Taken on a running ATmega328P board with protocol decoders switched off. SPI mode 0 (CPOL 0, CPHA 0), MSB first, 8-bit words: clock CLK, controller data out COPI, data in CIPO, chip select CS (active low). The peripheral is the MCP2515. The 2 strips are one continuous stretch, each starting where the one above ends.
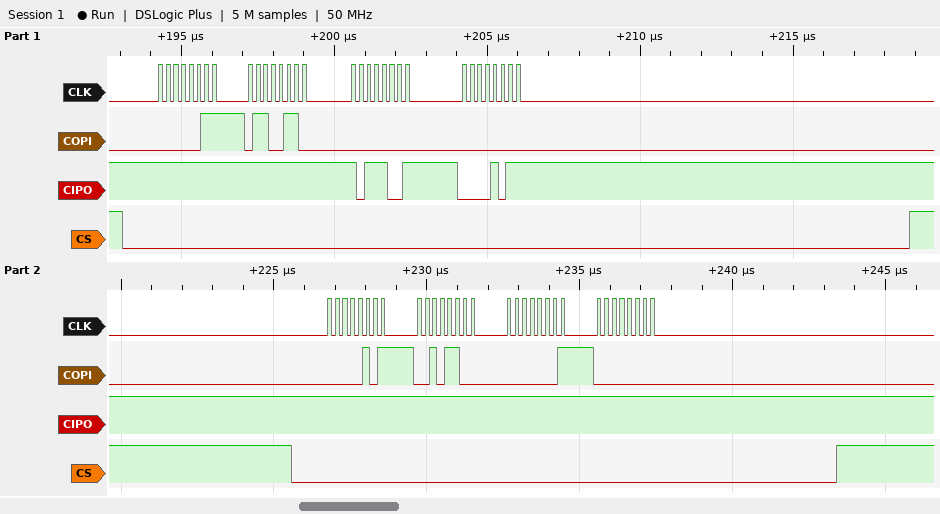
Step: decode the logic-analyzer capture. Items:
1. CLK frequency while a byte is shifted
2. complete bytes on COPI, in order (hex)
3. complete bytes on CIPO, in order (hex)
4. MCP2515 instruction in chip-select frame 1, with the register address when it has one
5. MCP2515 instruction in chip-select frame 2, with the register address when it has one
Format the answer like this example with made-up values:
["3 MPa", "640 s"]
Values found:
["4 MHz", "0x03 0x66 0x00 0x00 0x05 0x2C 0x01 0x00", "0xFF 0xFF 0xB9 0x0B 0xFF 0xFF 0xFF 0xFF", "READ 0x66", "BIT MODIFY 0x2C"]
